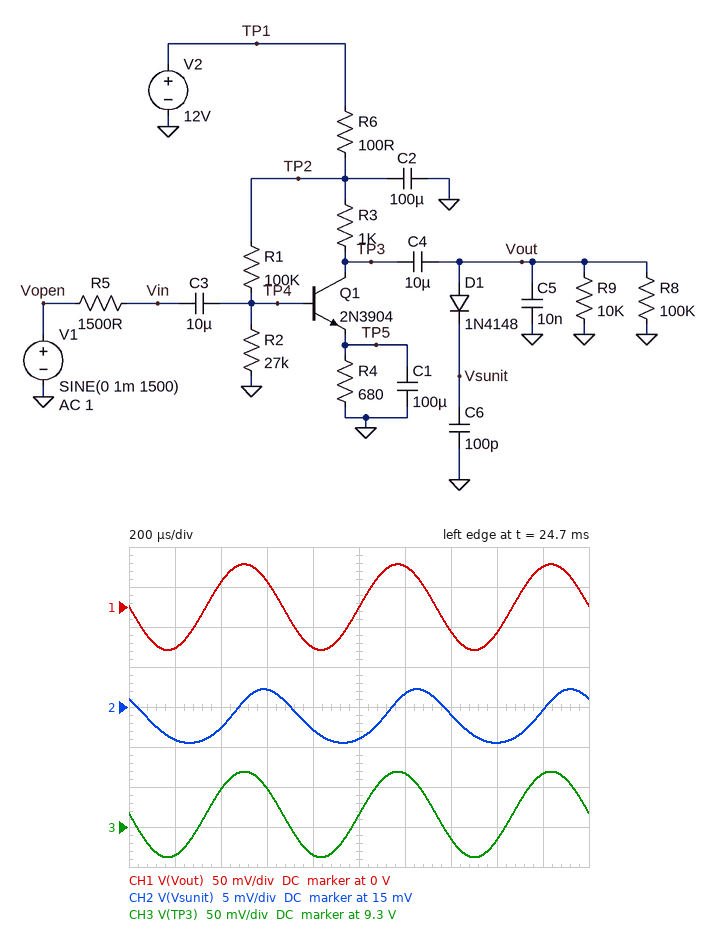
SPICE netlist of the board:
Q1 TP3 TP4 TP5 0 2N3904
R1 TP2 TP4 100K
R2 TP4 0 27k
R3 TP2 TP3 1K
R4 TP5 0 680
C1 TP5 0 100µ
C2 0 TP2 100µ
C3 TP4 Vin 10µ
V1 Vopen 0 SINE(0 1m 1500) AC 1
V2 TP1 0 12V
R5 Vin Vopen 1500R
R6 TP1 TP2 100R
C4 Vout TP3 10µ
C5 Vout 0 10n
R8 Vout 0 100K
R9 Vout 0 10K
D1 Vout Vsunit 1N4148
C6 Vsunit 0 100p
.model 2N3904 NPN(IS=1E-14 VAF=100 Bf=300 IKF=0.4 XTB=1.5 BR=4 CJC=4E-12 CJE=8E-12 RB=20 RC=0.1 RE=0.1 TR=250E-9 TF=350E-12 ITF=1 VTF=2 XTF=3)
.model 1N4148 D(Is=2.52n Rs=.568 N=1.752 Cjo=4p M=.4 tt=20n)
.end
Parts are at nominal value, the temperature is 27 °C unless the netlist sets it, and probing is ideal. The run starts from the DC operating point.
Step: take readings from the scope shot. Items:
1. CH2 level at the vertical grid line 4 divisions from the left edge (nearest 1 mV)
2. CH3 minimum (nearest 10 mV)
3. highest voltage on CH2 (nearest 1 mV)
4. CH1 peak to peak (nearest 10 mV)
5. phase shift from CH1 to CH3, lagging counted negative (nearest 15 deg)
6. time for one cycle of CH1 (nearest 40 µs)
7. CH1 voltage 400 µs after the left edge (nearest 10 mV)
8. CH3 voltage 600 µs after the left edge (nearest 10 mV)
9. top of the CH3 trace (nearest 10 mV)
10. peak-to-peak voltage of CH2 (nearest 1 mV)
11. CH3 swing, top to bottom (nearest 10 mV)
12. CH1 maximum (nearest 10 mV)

12 mV
9.26 V
17 mV
110 mV
0 deg
680 µs
30 mV
9.35 V
9.37 V
7 mV
110 mV
50 mV
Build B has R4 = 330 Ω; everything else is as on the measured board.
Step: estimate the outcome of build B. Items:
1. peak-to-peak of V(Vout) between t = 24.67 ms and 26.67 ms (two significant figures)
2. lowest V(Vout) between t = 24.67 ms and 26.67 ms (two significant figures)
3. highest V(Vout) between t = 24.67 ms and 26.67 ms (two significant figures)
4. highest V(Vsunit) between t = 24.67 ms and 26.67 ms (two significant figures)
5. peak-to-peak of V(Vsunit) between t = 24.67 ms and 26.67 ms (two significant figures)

150 mV
-76 mV
75 mV
30 mV
8.9 mV
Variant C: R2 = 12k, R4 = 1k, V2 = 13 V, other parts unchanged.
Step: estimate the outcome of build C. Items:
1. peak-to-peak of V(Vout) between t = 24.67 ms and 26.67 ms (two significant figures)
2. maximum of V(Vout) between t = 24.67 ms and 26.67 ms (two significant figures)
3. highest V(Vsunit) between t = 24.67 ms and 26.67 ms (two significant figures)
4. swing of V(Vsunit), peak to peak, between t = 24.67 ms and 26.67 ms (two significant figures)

39 mV
19 mV
3.2 mV
2.6 mV
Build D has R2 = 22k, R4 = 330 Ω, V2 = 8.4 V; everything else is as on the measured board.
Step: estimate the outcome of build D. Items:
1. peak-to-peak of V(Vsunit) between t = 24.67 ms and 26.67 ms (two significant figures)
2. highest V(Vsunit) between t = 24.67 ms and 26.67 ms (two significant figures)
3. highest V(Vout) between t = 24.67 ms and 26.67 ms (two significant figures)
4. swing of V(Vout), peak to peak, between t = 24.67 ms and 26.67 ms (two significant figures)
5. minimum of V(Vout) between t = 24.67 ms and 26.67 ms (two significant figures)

6.0 mV
14 mV
47 mV
94 mV
-47 mV
